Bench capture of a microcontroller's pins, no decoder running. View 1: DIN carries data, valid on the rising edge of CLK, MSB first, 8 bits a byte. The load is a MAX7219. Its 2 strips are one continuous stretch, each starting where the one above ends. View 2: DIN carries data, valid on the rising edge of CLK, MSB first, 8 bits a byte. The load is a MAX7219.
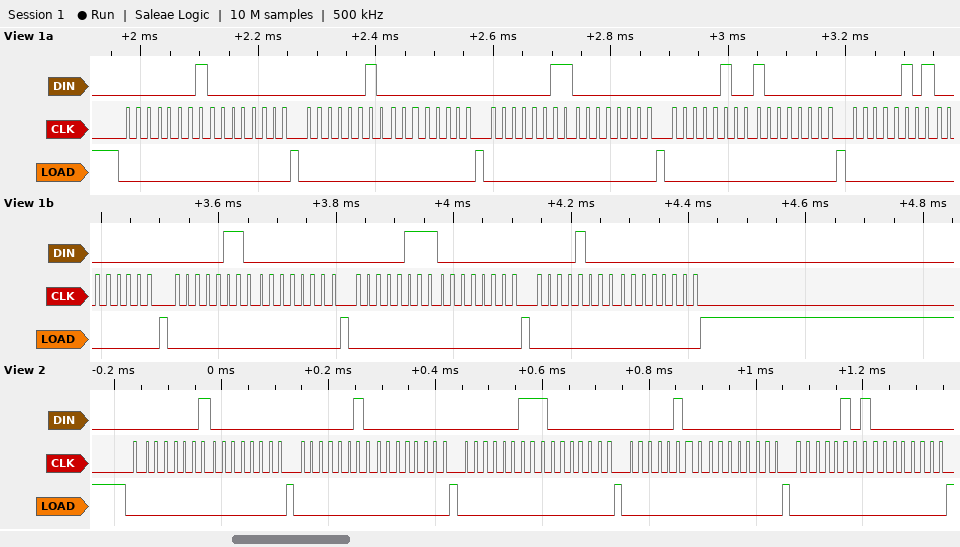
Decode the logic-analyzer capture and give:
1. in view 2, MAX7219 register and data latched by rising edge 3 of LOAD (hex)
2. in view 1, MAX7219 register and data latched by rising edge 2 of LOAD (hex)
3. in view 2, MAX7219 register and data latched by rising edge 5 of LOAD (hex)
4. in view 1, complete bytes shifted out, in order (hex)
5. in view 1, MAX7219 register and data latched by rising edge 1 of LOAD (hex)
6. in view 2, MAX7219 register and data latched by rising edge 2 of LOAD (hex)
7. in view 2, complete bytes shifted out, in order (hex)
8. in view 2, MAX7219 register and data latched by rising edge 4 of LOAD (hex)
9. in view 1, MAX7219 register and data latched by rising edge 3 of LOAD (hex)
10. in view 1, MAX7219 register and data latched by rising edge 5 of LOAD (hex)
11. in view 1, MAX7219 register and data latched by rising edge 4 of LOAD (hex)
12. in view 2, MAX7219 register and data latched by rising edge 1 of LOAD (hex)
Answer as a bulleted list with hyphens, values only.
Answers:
- register 0x3, data 0x80
- register 0x2, data 0x00
- register 0x5, data 0x00
- 0x01 0x00 0x02 0x00 0x03 0x00 0x04 0x80 0x05 0x00 0x06 0x00 0x07 0x00 0x08 0x00
- register 0x1, data 0x00
- register 0x2, data 0x00
- 01 00 02 00 03 80 04 00 05 00
- register 0x4, data 0x00
- register 0x3, data 0x00
- register 0x5, data 0x00
- register 0x4, data 0x80
- register 0x1, data 0x00
